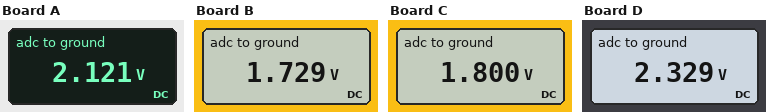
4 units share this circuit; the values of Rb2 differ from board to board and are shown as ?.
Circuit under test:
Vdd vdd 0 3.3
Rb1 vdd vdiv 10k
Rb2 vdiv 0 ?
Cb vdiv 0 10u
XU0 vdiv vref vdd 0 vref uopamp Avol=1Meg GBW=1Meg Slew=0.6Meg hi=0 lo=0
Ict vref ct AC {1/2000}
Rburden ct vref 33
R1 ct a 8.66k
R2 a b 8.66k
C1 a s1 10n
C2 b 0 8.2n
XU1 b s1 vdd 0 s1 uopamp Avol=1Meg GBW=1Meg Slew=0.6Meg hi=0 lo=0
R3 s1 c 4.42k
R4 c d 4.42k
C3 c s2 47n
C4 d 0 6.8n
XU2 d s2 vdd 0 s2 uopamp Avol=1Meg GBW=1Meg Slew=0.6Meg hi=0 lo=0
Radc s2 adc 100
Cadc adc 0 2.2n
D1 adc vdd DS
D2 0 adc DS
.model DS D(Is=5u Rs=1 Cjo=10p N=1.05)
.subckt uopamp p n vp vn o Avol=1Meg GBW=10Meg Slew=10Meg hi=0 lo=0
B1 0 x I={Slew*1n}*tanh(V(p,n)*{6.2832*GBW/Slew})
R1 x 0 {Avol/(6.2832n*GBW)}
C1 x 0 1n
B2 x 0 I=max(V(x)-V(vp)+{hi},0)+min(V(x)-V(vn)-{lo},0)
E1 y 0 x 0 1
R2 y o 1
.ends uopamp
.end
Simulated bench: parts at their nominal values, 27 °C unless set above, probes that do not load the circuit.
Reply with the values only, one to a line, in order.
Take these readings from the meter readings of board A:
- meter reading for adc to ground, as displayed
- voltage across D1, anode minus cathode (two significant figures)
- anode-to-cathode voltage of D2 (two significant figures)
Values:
2.121 V
-1.2 V
-2.1 V
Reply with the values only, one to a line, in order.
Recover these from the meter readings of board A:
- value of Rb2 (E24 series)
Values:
18 kΩ
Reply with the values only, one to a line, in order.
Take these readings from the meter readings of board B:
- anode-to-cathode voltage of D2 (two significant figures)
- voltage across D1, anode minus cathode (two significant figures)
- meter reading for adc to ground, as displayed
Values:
-1.7 V
-1.6 V
1.729 V
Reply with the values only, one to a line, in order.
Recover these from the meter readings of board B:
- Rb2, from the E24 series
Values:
11 kΩ
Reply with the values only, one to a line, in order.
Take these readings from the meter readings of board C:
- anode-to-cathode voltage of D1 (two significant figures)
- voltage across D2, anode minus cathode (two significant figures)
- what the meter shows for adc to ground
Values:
-1.5 V
-1.8 V
1.800 V
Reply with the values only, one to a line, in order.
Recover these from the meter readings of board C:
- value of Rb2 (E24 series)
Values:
12 kΩ
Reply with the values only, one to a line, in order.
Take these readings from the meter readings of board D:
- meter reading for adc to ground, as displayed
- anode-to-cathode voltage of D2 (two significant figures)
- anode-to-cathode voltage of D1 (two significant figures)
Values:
2.329 V
-2.3 V
-970 mV
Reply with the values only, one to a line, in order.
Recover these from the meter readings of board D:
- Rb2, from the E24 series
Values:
24 kΩ
